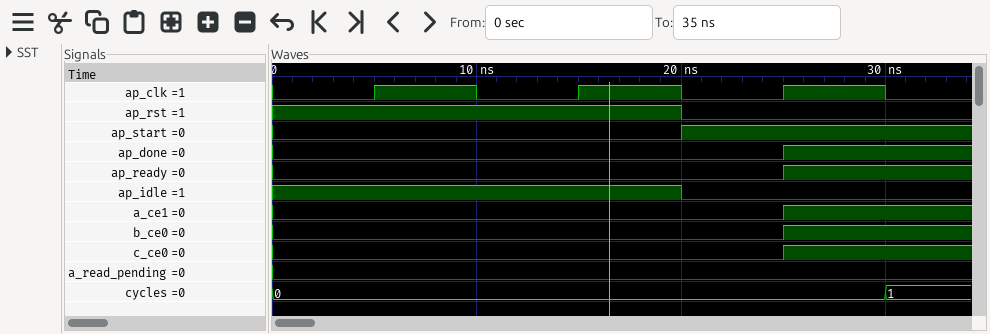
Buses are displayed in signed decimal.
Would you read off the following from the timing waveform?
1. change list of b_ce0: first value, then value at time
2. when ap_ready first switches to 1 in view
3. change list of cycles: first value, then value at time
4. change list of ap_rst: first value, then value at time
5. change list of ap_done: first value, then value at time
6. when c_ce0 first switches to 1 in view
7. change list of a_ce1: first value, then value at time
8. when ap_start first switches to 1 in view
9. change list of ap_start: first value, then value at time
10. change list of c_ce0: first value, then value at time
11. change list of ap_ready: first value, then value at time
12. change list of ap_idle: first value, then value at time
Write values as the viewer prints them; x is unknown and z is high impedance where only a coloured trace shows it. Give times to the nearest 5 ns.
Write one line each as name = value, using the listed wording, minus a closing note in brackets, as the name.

change list of b_ce0: first value, then value at time = 0, 1 at 25 ns
when ap_ready first switches to 1 in view = 25 ns
change list of cycles: first value, then value at time = 0, 1 at 30 ns
change list of ap_rst: first value, then value at time = 1, 0 at 20 ns
change list of ap_done: first value, then value at time = 0, 1 at 25 ns
when c_ce0 first switches to 1 in view = 25 ns
change list of a_ce1: first value, then value at time = 0, 1 at 25 ns
when ap_start first switches to 1 in view = 20 ns
change list of ap_start: first value, then value at time = 0, 1 at 20 ns
change list of c_ce0: first value, then value at time = 0, 1 at 25 ns
change list of ap_ready: first value, then value at time = 0, 1 at 25 ns
change list of ap_idle: first value, then value at time = 1, 0 at 20 ns
